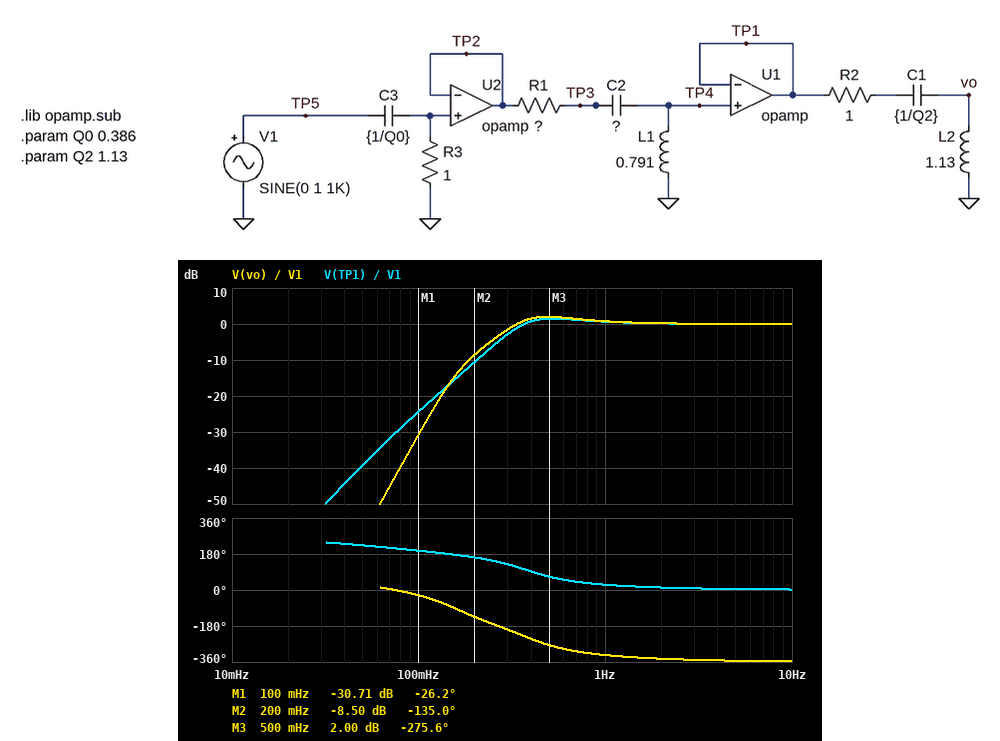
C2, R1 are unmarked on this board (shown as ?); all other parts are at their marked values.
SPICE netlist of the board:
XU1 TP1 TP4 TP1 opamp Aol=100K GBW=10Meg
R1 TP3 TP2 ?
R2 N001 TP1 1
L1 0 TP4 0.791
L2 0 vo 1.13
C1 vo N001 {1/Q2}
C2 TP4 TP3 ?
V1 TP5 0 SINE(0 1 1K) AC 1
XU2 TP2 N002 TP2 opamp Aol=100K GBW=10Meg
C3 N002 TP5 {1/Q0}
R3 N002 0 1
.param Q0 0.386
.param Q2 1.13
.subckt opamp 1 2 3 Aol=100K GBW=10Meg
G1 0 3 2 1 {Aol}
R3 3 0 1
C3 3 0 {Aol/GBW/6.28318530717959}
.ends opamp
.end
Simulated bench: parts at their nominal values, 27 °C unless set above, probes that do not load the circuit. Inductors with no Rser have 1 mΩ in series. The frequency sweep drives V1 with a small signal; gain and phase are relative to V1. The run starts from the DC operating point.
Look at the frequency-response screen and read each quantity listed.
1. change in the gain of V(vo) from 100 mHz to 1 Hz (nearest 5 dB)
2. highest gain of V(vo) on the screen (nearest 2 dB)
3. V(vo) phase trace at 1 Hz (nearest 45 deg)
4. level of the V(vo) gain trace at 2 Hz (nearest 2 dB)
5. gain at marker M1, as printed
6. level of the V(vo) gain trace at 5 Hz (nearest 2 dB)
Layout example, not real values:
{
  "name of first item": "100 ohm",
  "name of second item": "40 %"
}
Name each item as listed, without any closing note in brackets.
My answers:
{
  "change in the gain of V(vo) from 100 mHz to 1 Hz": "30 dB",
  "highest gain of V(vo) on the screen": "2 dB",
  "V(vo) phase trace at 1 Hz": "-315 deg",
  "level of the V(vo) gain trace at 2 Hz": "0 dB",
  "gain at marker M1, as printed": "-30.71 dB",
  "level of the V(vo) gain trace at 5 Hz": "0 dB"
}
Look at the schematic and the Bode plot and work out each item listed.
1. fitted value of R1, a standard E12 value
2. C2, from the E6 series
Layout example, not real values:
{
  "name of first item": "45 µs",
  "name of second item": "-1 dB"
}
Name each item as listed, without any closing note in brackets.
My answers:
{
  "fitted value of R1, a standard E12 value": "1.8 Ω",
  "C2, from the E6 series": "220 mF"
}
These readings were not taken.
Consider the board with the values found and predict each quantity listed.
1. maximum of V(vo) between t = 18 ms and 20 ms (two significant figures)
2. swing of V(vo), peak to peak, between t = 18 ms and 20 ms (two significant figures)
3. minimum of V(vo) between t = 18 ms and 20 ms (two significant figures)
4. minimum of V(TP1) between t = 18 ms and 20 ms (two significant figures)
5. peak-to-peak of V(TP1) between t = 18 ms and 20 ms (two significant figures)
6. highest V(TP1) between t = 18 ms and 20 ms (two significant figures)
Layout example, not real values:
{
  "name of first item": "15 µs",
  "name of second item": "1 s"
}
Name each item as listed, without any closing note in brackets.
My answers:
{
  "maximum of V(vo) between t = 18 ms and 20 ms": "1.0 V",
  "swing of V(vo), peak to peak, between t = 18 ms and 20 ms": "2.0 V",
  "minimum of V(vo) between t = 18 ms and 20 ms": "-1.0 V",
  "minimum of V(TP1) between t = 18 ms and 20 ms": "-1.0 V",
  "peak-to-peak of V(TP1) between t = 18 ms and 20 ms": "2.0 V",
  "highest V(TP1) between t = 18 ms and 20 ms": "1.0 V"
}
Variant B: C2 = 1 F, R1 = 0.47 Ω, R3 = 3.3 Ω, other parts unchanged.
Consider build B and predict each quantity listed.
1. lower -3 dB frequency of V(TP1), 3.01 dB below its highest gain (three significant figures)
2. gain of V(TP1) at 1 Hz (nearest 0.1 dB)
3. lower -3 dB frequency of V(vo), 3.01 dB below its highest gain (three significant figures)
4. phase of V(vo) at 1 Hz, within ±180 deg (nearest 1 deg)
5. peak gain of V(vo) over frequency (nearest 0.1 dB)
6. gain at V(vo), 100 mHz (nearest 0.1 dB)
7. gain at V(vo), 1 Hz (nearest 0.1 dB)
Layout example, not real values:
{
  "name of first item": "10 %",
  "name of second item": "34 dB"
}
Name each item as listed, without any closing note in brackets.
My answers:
{
  "lower -3 dB frequency of V(TP1), 3.01 dB below its highest gain": "153 mHz",
  "gain of V(TP1) at 1 Hz": "0.2 dB",
  "lower -3 dB frequency of V(vo), 3.01 dB below its highest gain": "159 mHz",
  "phase of V(vo) at 1 Hz, within ±180 deg": "15 deg",
  "peak gain of V(vo) over frequency": "7.8 dB",
  "gain at V(vo), 100 mHz": "-14.1 dB",
  "gain at V(vo), 1 Hz": "0.4 dB"
}
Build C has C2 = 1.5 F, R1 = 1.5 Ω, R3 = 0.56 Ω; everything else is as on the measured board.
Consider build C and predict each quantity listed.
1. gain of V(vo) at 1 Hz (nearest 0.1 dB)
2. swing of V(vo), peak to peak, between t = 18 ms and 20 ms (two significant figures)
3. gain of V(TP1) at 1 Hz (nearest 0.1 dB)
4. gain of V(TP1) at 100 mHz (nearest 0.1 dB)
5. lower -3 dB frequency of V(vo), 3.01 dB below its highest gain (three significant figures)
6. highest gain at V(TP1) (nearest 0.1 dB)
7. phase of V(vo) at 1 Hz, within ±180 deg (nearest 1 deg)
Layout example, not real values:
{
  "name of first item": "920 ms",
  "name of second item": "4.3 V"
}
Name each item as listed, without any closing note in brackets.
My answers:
{
  "gain of V(vo) at 1 Hz": "-0.1 dB",
  "swing of V(vo), peak to peak, between t = 18 ms and 20 ms": "2.0 V",
  "gain of V(TP1) at 1 Hz": "-0.3 dB",
  "gain of V(TP1) at 100 mHz": "-13.6 dB",
  "lower -3 dB frequency of V(vo), 3.01 dB below its highest gain": "203 mHz",
  "highest gain at V(TP1)": "0 dB",
  "phase of V(vo) at 1 Hz, within ±180 deg": "32 deg"
}
